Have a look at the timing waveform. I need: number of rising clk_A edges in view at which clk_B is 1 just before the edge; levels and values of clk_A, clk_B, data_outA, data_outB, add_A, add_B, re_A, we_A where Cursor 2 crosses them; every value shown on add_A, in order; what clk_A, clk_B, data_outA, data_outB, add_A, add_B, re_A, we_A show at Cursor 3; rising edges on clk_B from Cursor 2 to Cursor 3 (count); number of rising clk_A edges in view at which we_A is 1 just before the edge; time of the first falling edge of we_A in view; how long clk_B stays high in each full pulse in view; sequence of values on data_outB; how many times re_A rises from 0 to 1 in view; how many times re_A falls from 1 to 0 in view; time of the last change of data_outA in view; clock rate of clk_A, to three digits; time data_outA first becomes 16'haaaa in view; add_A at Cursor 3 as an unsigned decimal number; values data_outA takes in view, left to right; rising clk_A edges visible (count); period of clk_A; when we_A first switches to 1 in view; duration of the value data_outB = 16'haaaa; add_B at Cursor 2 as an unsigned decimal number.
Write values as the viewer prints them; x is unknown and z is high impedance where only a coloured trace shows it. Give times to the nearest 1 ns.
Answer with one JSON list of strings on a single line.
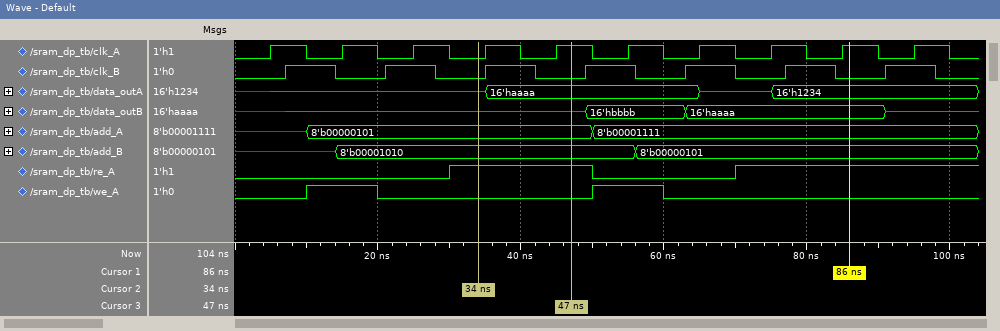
["4", "clk_A=0, clk_B=0, data_outA=z, data_outB=z, add_A=8'b00000101, add_B=8'b00001010, re_A=1, we_A=0", "x, 8'b00000101, 8'b00001111", "clk_A=1, clk_B=0, data_outA=16'haaaa, data_outB=z, add_A=8'b00000101, add_B=8'b00001010, re_A=1, we_A=0", "1", "2", "20 ns", "7 ns, 7 ns, 7 ns, 7 ns, 7 ns, 7 ns, 7 ns", "x, z, 16'hbbbb, 16'haaaa, z", "2", "1", "75 ns", "100 MHz", "35 ns", "5", "x, z, 16'haaaa, z, 16'h1234", "10", "10 ns", "10 ns", "28 ns", "10"]
